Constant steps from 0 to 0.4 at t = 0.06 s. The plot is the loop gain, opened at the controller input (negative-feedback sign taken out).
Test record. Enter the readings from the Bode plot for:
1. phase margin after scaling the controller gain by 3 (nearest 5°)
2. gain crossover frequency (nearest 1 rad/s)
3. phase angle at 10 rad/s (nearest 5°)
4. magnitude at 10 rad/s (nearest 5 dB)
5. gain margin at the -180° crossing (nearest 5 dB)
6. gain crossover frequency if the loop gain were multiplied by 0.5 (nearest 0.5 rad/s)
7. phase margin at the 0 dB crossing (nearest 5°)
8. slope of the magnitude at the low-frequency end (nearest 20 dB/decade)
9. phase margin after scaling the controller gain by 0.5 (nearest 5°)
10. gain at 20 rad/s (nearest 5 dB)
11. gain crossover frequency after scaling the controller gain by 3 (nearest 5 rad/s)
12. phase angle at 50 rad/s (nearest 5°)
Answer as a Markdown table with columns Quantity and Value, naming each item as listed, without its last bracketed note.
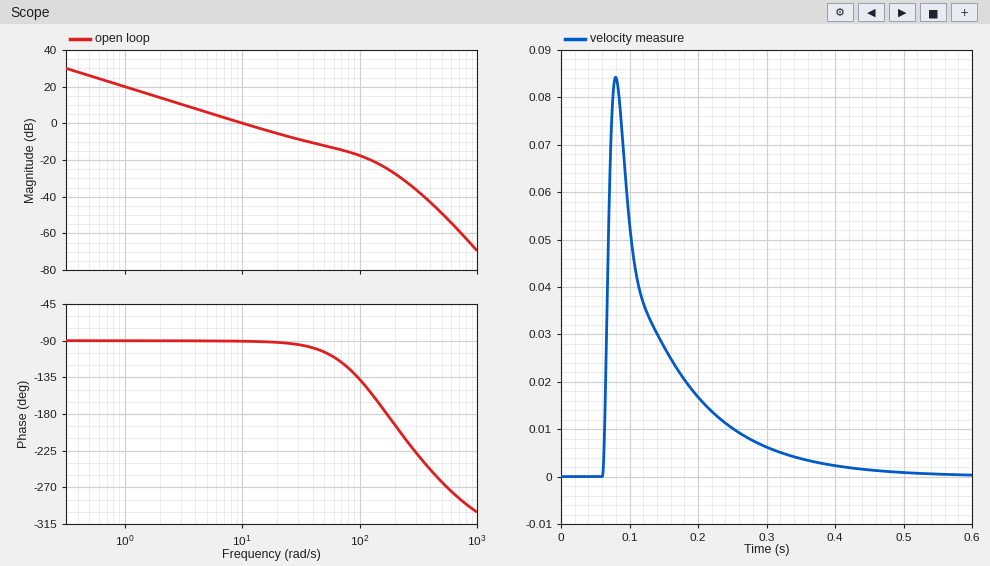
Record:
| Quantity | Value |
|---|---|
| phase margin after scaling the controller gain by 3 | 85° |
| gain crossover frequency | 10 rad/s |
| phase angle at 10 rad/s | -90° |
| magnitude at 10 rad/s | 0 dB |
| gain margin at the -180° crossing | 25 dB |
| gain crossover frequency if the loop gain were multiplied by 0.5 | 5.0 rad/s |
| phase margin at the 0 dB crossing | 90° |
| slope of the magnitude at the low-frequency end | -20 dB/decade |
| phase margin after scaling the controller gain by 0.5 | 90° |
| gain at 20 rad/s | -5 dB |
| gain crossover frequency after scaling the controller gain by 3 | 35 rad/s |
| phase angle at 50 rad/s | -105° |
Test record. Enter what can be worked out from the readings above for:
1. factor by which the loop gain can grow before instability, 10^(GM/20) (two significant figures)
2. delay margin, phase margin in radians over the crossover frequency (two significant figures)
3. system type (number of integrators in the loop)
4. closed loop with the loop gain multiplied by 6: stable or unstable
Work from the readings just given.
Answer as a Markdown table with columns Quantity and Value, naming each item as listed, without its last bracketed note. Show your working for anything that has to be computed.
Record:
| Quantity | Value |
|---|---|
| factor by which the loop gain can grow before instability, 10^(GM/20) | 10^(25 / 20) = 18 |
| delay margin, phase margin in radians over the crossover frequency | 90 × π / 180 / 10 = 0.16 s |
| system type | 1 |
| closed loop with the loop gain multiplied by 6: stable or unstable | stable |
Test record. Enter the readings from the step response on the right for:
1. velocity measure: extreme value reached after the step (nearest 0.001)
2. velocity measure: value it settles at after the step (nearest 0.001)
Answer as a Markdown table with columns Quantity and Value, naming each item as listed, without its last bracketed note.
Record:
| Quantity | Value |
|---|---|
| velocity measure: extreme value reached after the step | 0.084 |
| velocity measure: value it settles at after the step | 0.000 |
